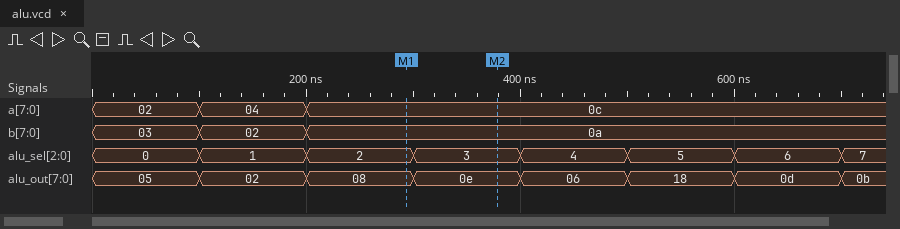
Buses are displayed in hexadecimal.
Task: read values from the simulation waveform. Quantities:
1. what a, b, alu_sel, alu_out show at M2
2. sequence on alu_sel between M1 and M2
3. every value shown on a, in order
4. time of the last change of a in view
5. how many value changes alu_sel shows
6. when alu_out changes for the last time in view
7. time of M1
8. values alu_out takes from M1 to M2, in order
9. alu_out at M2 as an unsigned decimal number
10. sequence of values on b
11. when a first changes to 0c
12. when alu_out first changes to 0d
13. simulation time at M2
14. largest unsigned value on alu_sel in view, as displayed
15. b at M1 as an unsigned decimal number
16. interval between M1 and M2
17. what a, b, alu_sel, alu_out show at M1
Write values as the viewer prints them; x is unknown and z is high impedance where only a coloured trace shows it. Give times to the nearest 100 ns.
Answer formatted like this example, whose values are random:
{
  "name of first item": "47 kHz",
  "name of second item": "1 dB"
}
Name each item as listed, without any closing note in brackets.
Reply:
{
  "what a, b, alu_sel, alu_out show at M2": "a=0c, b=0a, alu_sel=3, alu_out=0e",
  "sequence on alu_sel between M1 and M2": "2, 3",
  "every value shown on a, in order": "02, 04, 0c",
  "time of the last change of a in view": "200 ns",
  "how many value changes alu_sel shows": "7",
  "when alu_out changes for the last time in view": "700 ns",
  "time of M1": "300 ns",
  "values alu_out takes from M1 to M2, in order": "08, 0e",
  "alu_out at M2 as an unsigned decimal number": "14",
  "sequence of values on b": "03, 02, 0a",
  "when a first changes to 0c": "200 ns",
  "when alu_out first changes to 0d": "600 ns",
  "simulation time at M2": "400 ns",
  "largest unsigned value on alu_sel in view, as displayed": "7",
  "b at M1 as an unsigned decimal number": "10",
  "interval between M1 and M2": "100 ns",
  "what a, b, alu_sel, alu_out show at M1": "a=0c, b=0a, alu_sel=2, alu_out=08"
}
